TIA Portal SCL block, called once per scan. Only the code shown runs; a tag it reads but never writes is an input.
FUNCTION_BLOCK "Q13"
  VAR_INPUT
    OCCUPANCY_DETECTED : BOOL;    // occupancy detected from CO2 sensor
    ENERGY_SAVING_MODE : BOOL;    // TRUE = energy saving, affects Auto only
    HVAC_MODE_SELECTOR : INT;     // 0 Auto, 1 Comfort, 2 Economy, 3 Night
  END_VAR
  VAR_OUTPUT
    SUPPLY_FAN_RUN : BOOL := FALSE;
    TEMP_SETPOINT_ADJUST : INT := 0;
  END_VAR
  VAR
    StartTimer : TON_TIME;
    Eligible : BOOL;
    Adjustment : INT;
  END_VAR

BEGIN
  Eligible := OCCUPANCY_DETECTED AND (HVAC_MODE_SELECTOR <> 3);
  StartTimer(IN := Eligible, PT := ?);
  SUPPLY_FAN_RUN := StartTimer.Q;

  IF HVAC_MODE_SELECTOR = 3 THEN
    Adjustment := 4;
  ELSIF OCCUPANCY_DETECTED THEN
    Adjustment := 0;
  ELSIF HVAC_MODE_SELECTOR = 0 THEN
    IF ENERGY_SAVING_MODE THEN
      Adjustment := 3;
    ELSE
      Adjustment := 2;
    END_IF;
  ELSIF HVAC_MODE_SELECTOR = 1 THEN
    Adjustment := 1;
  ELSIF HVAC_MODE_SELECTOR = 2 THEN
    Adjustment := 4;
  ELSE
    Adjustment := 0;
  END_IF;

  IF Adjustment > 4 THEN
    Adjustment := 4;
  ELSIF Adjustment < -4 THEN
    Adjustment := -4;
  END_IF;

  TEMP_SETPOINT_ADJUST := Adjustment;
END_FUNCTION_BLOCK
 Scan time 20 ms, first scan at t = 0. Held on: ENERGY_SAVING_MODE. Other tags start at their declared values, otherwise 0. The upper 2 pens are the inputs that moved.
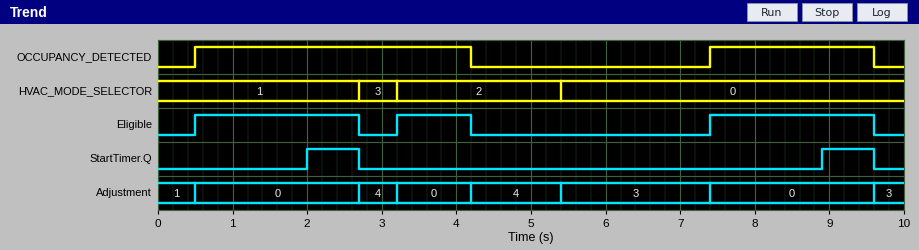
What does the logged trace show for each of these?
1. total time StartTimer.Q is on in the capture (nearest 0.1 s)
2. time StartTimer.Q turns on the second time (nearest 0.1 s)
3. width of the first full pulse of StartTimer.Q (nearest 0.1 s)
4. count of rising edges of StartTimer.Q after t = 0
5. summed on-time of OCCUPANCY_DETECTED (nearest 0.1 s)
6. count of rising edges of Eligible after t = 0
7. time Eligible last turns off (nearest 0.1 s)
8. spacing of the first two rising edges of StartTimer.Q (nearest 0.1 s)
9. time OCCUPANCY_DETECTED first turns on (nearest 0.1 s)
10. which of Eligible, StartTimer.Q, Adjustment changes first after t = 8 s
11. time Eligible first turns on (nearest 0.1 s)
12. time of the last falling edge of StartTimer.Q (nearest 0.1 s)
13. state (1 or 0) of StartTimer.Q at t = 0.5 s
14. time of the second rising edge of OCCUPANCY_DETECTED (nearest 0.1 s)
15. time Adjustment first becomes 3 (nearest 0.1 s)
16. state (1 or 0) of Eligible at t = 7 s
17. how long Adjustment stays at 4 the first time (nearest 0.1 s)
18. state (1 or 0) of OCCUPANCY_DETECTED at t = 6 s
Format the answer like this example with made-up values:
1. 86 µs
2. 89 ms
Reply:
1. 1.4 s
2. 8.9 s
3. 0.7 s
4. 2
5. 5.9 s
6. 3
7. 9.6 s
8. 6.9 s
9. 0.5 s
10. StartTimer.Q
11. 0.5 s
12. 9.6 s
13. 0
14. 7.4 s
15. 5.4 s
16. 0
17. 0.5 s
18. 0
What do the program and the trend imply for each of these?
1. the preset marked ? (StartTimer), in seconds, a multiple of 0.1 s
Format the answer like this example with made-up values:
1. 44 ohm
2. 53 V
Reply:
1. 1.5 s
